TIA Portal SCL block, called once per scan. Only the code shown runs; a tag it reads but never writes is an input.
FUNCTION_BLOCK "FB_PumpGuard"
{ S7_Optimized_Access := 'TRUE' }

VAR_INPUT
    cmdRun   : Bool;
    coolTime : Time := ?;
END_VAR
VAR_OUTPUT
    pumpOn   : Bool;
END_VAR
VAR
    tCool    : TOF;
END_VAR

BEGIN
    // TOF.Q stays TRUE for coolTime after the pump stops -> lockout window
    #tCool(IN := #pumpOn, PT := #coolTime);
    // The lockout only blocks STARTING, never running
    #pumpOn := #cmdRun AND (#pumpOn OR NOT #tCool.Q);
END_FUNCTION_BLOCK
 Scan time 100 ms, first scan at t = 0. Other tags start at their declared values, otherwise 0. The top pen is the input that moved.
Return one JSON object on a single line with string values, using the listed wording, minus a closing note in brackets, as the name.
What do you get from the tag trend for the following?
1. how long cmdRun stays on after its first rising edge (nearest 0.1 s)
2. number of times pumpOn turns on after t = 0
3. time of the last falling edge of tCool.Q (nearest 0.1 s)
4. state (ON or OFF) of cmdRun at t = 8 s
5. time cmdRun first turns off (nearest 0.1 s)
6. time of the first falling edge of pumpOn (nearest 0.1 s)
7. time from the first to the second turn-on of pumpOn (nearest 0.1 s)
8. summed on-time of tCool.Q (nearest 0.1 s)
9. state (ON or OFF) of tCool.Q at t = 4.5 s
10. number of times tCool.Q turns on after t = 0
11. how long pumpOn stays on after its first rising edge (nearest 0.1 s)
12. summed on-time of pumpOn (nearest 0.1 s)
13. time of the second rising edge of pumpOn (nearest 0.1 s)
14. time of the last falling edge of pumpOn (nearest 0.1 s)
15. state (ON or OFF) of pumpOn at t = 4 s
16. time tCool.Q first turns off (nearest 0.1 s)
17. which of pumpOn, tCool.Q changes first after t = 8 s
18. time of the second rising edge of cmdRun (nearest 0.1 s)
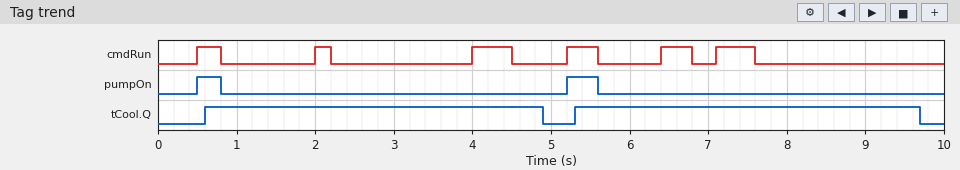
{"how long cmdRun stays on after its first rising edge": "0.3 s", "number of times pumpOn turns on after t = 0": "2", "time of the last falling edge of tCool.Q": "9.7 s", "state (ON or OFF) of cmdRun at t = 8 s": "OFF", "time cmdRun first turns off": "0.8 s", "time of the first falling edge of pumpOn": "0.8 s", "time from the first to the second turn-on of pumpOn": "4.7 s", "summed on-time of tCool.Q": "8.7 s", "state (ON or OFF) of tCool.Q at t = 4.5 s": "ON", "number of times tCool.Q turns on after t = 0": "2", "how long pumpOn stays on after its first rising edge": "0.3 s", "summed on-time of pumpOn": "0.7 s", "time of the second rising edge of pumpOn": "5.2 s", "time of the last falling edge of pumpOn": "5.6 s", "state (ON or OFF) of pumpOn at t = 4 s": "OFF", "time tCool.Q first turns off": "4.9 s", "which of pumpOn, tCool.Q changes first after t = 8 s": "tCool.Q", "time of the second rising edge of cmdRun": "2.0 s"}
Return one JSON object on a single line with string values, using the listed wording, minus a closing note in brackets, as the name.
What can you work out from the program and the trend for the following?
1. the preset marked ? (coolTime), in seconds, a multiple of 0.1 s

{"the preset marked ? (coolTime), in seconds, a multiple of 0.1 s": "4.0 s"}
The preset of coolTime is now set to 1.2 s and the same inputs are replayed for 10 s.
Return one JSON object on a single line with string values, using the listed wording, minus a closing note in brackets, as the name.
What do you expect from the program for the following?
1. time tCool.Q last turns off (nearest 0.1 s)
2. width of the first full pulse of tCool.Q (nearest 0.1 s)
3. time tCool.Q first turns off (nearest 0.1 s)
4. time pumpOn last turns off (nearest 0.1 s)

{"time tCool.Q last turns off": "8.1 s", "width of the first full pulse of tCool.Q": "1.5 s", "time tCool.Q first turns off": "2.1 s", "time pumpOn last turns off": "6.8 s"}
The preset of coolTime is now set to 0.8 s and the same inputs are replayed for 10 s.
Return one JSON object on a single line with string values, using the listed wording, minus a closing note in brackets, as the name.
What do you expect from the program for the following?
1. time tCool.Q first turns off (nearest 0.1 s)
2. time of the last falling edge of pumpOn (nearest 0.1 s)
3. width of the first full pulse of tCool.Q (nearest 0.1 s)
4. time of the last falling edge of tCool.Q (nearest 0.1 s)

{"time tCool.Q first turns off": "1.7 s", "time of the last falling edge of pumpOn": "6.8 s", "width of the first full pulse of tCool.Q": "1.1 s", "time of the last falling edge of tCool.Q": "7.7 s"}
